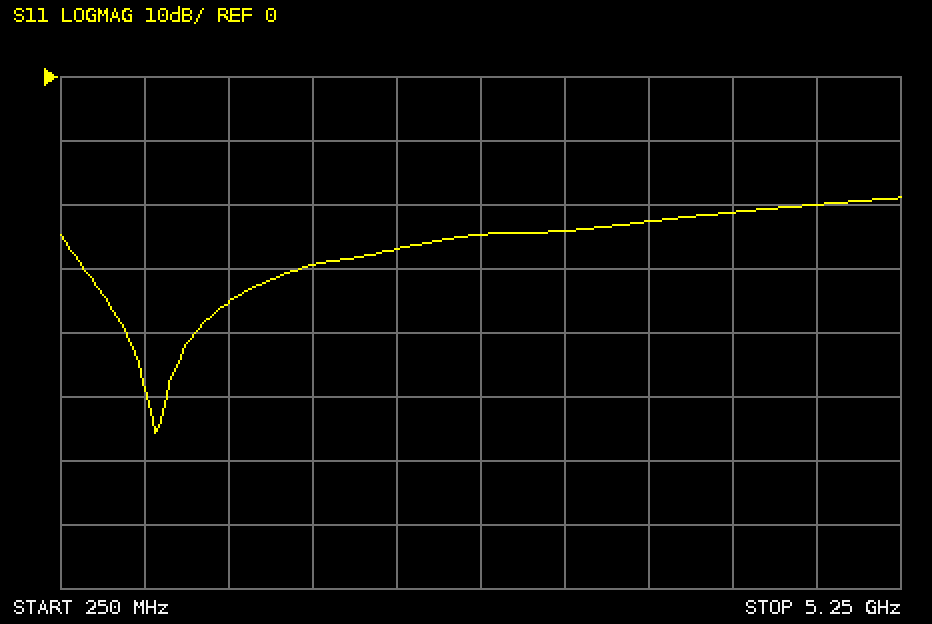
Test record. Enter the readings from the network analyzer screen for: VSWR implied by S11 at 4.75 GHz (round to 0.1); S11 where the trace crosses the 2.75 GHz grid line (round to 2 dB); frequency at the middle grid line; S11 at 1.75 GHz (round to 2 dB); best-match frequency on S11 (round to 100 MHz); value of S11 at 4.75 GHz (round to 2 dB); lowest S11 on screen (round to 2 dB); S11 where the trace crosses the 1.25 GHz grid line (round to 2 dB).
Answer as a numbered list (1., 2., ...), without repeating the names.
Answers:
1. 1.2
2. -24 dB
3. 2.75 GHz
4. -30 dB
5. 800 MHz
6. -20 dB
7. -56 dB
8. -36 dB
